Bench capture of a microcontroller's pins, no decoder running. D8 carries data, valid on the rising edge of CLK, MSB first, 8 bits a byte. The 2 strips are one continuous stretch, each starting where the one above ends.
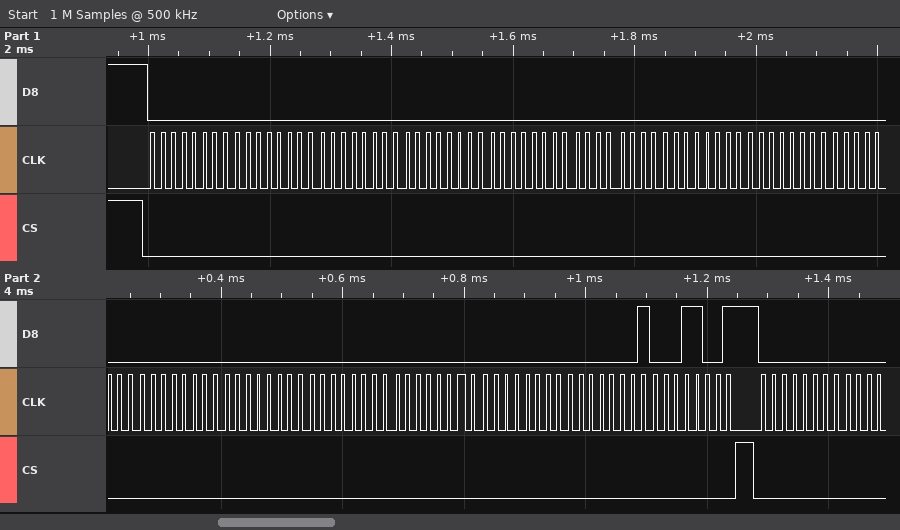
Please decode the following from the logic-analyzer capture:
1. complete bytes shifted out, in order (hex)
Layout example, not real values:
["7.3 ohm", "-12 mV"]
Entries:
["00 00 00 00 00 00 00 00 00 00 00 00 00 00 01 19 00"]
